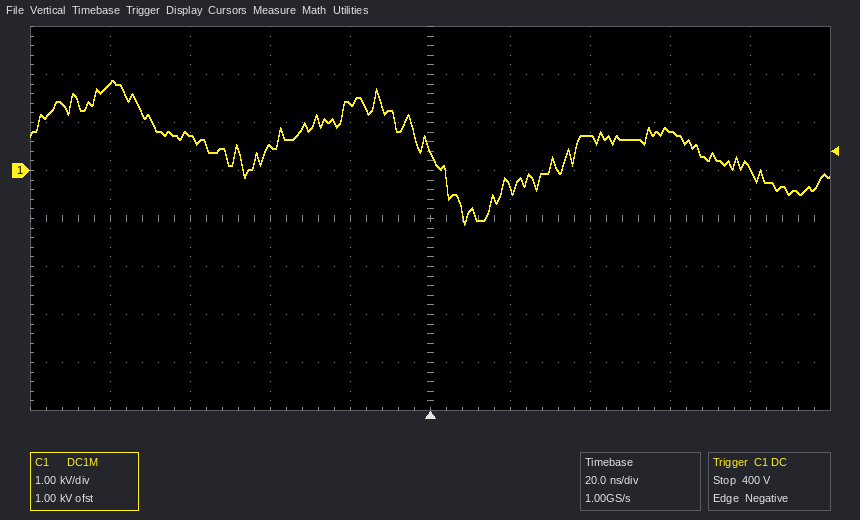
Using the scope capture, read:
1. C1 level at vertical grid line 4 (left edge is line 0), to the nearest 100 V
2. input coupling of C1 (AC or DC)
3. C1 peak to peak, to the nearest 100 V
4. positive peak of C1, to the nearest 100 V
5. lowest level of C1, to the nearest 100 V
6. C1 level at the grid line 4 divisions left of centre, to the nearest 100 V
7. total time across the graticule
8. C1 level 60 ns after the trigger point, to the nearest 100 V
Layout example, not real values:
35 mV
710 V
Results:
1.4 kV
DC
3.0 kV
1.9 kV
-1.1 kV
1.8 kV
200 ns
800 V
